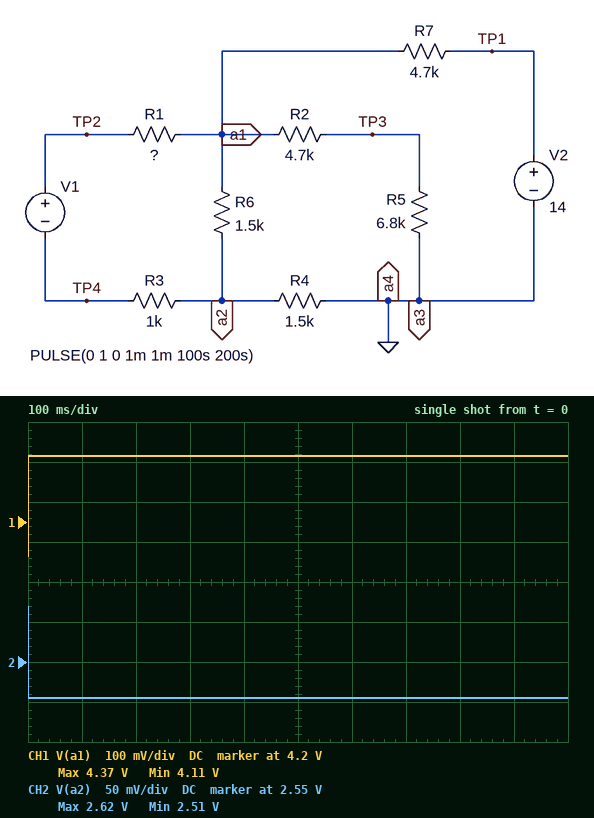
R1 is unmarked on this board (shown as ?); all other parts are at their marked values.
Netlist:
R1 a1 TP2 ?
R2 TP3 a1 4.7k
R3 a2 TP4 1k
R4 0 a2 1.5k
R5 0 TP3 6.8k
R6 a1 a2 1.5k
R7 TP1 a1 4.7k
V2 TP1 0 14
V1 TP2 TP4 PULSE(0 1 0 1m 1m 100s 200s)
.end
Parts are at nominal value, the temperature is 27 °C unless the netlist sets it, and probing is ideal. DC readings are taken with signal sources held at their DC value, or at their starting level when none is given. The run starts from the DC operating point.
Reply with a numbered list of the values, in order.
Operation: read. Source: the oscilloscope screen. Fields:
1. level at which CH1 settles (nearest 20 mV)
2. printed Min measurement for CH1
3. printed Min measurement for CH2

1. 4.36 V
2. 4.11 V
3. 2.51 V
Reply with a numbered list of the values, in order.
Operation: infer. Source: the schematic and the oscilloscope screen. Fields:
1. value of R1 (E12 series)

1. 1 kΩ
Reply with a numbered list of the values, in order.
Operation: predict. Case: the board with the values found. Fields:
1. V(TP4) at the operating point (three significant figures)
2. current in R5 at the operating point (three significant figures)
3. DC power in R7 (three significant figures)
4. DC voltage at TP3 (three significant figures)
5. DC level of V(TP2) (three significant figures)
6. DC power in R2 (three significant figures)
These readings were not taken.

1. 3.37 V
2. 358 µA
3. 20.8 mW
4. 2.43 V
5. 3.37 V
6. 602 µW
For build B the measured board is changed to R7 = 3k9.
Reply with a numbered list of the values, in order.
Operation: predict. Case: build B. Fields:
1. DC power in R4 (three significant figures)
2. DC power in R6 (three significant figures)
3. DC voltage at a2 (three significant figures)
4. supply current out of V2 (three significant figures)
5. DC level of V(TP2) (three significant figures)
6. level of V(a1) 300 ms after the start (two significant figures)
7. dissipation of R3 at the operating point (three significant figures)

1. 5.90 mW
2. 1.93 mW
3. 2.98 V
4. 2.39 mA
5. 3.83 V
6. 4.9 V
7. 723 µW
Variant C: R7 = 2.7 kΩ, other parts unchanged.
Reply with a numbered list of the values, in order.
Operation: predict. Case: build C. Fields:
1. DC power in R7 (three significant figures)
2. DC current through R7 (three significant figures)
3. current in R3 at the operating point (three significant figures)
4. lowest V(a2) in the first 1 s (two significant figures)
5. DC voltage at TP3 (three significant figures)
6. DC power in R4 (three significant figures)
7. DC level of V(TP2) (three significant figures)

1. 24.4 mW
2. 3.01 mA
3. 1.07 mA
4. 3.6 V
5. 3.48 V
6. 9.34 mW
7. 4.81 V
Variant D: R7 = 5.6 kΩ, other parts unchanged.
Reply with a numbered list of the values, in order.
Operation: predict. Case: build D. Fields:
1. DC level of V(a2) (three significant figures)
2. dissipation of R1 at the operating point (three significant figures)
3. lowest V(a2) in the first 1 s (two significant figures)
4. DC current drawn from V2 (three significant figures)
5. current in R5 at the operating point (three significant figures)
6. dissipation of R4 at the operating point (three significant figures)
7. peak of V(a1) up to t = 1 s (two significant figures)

1. 2.31 V
2. 434 µW
3. 2.2 V
4. 1.85 mA
5. 315 µA
6. 3.55 mW
7. 3.9 V
